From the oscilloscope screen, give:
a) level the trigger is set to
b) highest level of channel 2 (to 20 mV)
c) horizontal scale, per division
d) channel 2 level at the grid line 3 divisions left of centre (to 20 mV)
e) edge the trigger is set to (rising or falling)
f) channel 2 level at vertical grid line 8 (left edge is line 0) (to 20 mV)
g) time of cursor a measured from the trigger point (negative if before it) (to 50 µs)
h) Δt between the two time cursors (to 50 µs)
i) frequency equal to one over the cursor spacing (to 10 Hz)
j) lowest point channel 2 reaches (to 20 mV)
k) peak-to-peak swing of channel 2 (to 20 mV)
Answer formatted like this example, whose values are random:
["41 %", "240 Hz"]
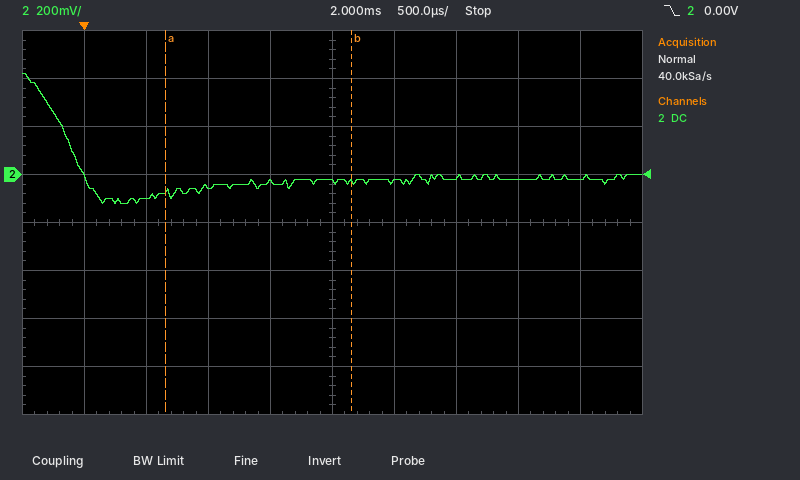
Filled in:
["0.00 V", "420 mV", "500 µs", "-100 mV", "falling", "-20 mV", "+650 µs", "1.50 ms", "670 Hz", "-120 mV", "540 mV"]
